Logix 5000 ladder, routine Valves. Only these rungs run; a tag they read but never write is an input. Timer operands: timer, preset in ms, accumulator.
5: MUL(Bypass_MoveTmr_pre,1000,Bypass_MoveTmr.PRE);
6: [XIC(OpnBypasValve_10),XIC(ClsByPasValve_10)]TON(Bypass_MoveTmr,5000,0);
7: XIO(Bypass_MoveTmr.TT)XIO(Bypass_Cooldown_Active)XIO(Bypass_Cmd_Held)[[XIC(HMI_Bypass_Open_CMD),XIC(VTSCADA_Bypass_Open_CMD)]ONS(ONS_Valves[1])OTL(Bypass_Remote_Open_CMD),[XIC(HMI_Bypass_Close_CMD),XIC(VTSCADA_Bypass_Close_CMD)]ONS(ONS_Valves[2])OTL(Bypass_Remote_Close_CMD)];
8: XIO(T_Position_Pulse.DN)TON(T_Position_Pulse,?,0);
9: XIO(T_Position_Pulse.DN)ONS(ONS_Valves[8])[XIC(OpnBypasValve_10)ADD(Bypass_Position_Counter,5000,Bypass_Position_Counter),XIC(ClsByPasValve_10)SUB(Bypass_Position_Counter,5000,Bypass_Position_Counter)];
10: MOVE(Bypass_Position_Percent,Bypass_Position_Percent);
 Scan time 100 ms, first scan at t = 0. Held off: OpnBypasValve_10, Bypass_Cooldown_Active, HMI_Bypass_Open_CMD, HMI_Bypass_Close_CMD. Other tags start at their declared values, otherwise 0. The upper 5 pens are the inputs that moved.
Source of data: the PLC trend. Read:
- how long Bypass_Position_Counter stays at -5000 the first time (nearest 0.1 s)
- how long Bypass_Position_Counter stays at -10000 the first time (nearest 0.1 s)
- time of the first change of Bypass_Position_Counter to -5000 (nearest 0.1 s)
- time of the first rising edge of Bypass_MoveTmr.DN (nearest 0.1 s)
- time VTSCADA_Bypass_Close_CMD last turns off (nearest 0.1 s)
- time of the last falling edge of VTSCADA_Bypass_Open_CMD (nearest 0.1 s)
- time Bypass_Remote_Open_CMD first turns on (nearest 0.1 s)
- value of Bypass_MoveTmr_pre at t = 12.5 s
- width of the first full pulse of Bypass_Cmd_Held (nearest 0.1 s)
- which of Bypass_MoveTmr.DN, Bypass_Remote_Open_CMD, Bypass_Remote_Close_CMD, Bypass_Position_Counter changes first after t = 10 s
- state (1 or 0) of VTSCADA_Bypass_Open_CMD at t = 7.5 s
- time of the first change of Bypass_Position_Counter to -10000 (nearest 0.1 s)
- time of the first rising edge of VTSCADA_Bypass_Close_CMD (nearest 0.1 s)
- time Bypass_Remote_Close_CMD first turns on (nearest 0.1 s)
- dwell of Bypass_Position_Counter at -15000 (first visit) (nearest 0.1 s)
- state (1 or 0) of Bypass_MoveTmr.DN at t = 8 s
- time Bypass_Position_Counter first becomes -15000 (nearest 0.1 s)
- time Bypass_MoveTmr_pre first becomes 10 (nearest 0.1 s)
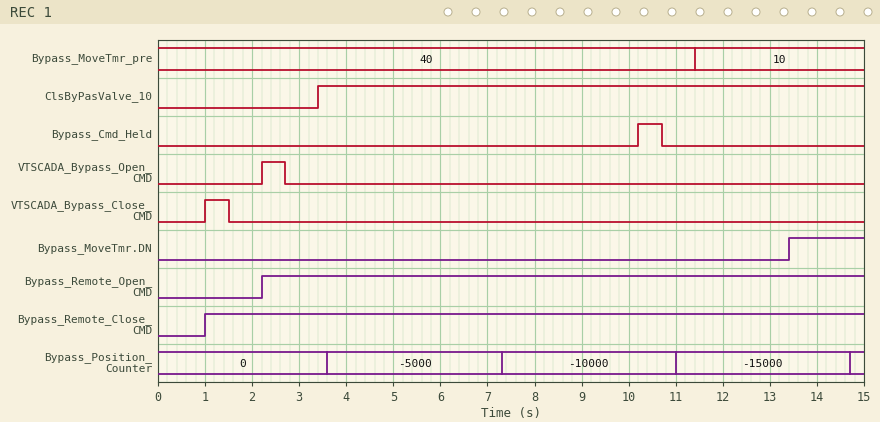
3.7 s
3.7 s
3.6 s
13.4 s
1.5 s
2.7 s
2.2 s
10
0.5 s
Bypass_Position_Counter
0
7.3 s
1.0 s
1.0 s
3.7 s
0
11.0 s
11.4 s
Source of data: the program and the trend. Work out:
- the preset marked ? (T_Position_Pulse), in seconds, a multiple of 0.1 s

3.5 s
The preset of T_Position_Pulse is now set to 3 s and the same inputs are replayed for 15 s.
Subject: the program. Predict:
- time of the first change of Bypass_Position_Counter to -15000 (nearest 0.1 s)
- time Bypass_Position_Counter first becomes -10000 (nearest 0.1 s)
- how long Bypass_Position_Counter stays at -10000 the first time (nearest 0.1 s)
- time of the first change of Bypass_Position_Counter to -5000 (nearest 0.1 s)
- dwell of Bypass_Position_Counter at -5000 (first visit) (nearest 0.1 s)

12.7 s
9.5 s
3.2 s
6.3 s
3.2 s
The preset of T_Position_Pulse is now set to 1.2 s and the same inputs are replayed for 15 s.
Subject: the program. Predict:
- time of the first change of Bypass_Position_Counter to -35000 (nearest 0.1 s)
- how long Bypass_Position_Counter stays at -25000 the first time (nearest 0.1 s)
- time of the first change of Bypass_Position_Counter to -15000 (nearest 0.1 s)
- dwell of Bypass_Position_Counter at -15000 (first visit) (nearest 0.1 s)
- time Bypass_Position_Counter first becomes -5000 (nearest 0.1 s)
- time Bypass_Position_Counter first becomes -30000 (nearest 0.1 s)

12.5 s
1.4 s
6.9 s
1.4 s
4.1 s
11.1 s
